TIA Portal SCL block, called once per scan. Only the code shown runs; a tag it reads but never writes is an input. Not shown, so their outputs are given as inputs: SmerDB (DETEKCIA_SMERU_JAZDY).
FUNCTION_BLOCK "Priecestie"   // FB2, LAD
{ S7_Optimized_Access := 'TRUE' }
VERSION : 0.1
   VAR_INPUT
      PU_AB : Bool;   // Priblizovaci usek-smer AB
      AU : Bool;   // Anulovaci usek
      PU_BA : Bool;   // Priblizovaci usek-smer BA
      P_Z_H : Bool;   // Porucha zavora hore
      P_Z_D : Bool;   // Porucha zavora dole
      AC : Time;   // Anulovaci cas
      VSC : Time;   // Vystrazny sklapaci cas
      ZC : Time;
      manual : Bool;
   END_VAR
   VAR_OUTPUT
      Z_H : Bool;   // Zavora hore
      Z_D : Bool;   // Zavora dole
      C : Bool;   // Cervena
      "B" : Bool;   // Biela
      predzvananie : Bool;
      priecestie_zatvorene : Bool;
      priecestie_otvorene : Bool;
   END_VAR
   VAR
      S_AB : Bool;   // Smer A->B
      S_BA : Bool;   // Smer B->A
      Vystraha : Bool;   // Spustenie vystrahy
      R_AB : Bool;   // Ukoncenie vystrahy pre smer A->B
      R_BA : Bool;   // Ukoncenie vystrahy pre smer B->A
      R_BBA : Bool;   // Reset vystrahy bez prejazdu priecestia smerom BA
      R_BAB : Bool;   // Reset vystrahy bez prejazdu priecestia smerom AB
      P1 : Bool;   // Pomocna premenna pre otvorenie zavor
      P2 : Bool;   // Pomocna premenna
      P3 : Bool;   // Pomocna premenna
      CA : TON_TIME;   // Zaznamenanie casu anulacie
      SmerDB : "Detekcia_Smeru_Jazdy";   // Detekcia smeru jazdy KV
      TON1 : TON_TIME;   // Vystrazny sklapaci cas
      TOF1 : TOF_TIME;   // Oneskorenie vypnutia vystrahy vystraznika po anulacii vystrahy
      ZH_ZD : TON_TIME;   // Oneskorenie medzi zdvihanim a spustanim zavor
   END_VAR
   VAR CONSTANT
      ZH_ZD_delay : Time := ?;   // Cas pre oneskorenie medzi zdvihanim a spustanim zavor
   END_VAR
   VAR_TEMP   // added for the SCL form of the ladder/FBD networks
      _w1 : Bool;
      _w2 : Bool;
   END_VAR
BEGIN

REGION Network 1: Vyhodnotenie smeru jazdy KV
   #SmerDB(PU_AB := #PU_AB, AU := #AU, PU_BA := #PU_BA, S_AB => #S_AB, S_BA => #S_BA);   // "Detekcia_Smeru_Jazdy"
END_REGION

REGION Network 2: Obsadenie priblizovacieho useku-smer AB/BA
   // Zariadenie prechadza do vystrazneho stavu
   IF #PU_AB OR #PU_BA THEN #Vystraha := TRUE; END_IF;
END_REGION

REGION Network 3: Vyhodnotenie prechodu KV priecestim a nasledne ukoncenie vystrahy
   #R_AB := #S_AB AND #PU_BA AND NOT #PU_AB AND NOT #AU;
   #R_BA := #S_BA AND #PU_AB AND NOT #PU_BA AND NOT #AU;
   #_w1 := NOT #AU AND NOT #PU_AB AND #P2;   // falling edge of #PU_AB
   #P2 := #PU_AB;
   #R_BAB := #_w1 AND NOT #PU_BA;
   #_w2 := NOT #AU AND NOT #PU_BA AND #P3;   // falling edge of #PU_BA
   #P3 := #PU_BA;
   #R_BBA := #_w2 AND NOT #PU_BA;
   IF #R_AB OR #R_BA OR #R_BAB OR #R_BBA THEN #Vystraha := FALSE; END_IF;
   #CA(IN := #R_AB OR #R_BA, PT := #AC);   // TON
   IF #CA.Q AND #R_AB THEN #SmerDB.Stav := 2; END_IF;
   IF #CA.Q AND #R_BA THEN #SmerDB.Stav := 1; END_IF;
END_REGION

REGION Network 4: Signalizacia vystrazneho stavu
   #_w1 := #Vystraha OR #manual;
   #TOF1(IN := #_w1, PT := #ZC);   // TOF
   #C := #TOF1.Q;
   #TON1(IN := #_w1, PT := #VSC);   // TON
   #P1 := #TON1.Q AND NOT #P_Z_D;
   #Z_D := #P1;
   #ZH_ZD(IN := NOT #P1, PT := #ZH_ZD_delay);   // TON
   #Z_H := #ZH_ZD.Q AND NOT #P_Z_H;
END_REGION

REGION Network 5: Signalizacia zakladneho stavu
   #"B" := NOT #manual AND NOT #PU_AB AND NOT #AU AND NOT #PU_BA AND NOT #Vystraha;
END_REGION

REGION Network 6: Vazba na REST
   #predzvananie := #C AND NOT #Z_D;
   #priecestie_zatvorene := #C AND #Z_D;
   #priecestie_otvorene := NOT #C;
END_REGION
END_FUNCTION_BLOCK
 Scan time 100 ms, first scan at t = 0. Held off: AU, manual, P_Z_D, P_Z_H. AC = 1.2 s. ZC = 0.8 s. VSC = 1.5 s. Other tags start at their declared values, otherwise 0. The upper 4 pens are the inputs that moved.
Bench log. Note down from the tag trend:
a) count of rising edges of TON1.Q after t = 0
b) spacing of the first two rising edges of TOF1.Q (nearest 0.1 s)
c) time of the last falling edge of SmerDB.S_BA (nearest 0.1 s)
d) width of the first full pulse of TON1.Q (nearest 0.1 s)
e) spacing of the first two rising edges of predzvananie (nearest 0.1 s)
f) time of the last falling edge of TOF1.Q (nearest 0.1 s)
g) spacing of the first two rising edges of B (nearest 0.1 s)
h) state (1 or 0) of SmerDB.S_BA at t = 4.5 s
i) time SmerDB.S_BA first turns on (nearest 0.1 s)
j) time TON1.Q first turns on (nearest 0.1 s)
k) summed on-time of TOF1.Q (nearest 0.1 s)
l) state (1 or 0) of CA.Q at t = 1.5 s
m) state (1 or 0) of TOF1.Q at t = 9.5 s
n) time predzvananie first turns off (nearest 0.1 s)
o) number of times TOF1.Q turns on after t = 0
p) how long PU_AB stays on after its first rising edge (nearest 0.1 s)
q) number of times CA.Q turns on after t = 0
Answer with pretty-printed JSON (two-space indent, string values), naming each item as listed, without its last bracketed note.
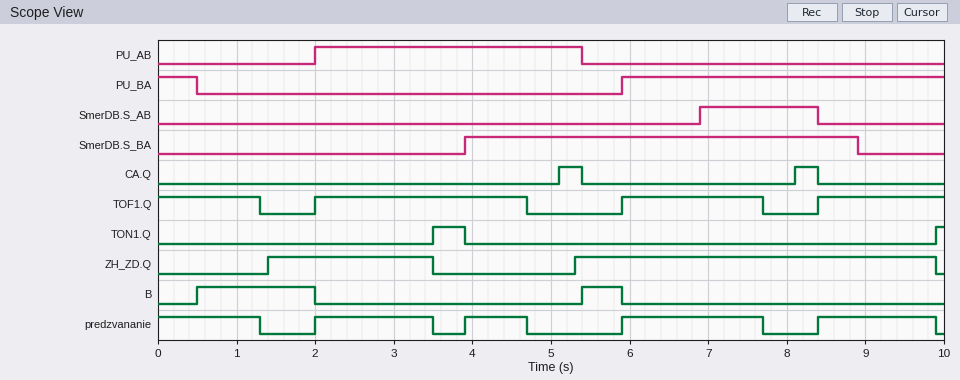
{
  "count of rising edges of TON1.Q after t = 0": "2",
  "spacing of the first two rising edges of TOF1.Q": "3.9 s",
  "time of the last falling edge of SmerDB.S_BA": "8.9 s",
  "width of the first full pulse of TON1.Q": "0.4 s",
  "spacing of the first two rising edges of predzvananie": "1.9 s",
  "time of the last falling edge of TOF1.Q": "7.7 s",
  "spacing of the first two rising edges of B": "4.9 s",
  "state (1 or 0) of SmerDB.S_BA at t = 4.5 s": "1",
  "time SmerDB.S_BA first turns on": "3.9 s",
  "time TON1.Q first turns on": "3.5 s",
  "summed on-time of TOF1.Q": "7.4 s",
  "state (1 or 0) of CA.Q at t = 1.5 s": "0",
  "state (1 or 0) of TOF1.Q at t = 9.5 s": "1",
  "time predzvananie first turns off": "1.3 s",
  "number of times TOF1.Q turns on after t = 0": "3",
  "how long PU_AB stays on after its first rising edge": "3.4 s",
  "number of times CA.Q turns on after t = 0": "2"
}
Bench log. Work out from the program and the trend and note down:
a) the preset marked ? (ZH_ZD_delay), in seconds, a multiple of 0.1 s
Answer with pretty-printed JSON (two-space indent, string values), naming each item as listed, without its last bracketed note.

{
  "the preset marked ? (ZH_ZD_delay), in seconds, a multiple of 0.1 s": "1.4 s"
}
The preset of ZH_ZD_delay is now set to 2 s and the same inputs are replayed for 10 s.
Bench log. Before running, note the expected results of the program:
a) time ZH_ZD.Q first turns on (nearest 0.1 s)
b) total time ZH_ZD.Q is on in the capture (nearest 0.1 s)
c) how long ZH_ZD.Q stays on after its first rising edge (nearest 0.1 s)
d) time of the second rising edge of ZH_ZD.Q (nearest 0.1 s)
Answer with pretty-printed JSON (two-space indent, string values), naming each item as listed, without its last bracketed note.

{
  "time ZH_ZD.Q first turns on": "2.0 s",
  "total time ZH_ZD.Q is on in the capture": "5.5 s",
  "how long ZH_ZD.Q stays on after its first rising edge": "1.5 s",
  "time of the second rising edge of ZH_ZD.Q": "5.9 s"
}
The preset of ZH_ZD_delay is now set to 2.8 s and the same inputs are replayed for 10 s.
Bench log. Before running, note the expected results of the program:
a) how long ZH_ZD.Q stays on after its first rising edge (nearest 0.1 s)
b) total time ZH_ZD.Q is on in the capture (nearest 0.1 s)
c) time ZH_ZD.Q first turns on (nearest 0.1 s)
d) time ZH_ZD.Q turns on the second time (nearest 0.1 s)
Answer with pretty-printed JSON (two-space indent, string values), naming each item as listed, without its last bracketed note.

{
  "how long ZH_ZD.Q stays on after its first rising edge": "0.7 s",
  "total time ZH_ZD.Q is on in the capture": "3.9 s",
  "time ZH_ZD.Q first turns on": "2.8 s",
  "time ZH_ZD.Q turns on the second time": "6.7 s"
}
